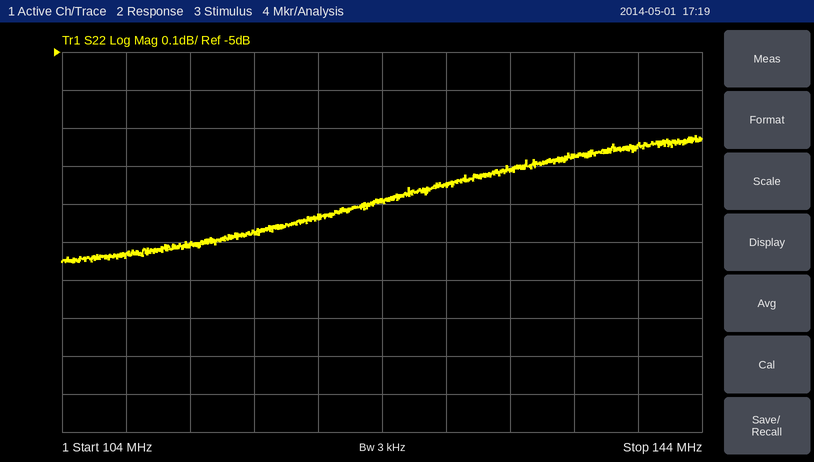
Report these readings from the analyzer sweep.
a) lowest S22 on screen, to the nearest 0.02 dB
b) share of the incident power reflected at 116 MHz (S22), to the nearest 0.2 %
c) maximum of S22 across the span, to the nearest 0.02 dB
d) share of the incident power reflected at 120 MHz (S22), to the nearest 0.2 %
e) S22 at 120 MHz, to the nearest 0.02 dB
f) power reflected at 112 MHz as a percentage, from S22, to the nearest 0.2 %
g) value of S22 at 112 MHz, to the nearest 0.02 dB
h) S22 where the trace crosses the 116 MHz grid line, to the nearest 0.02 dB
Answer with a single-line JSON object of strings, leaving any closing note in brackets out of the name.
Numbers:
{"lowest S22 on screen, to the nearest 0.02 dB": "-5.56 dB", "share of the incident power reflected at 116 MHz (S22), to the nearest 0.2 %": "28.4 %", "maximum of S22 across the span, to the nearest 0.02 dB": "-5.22 dB", "share of the incident power reflected at 120 MHz (S22), to the nearest 0.2 %": "28.6 %", "S22 at 120 MHz, to the nearest 0.02 dB": "-5.44 dB", "power reflected at 112 MHz as a percentage, from S22, to the nearest 0.2 %": "28.2 %", "value of S22 at 112 MHz, to the nearest 0.02 dB": "-5.50 dB", "S22 where the trace crosses the 116 MHz grid line, to the nearest 0.02 dB": "-5.48 dB"}
